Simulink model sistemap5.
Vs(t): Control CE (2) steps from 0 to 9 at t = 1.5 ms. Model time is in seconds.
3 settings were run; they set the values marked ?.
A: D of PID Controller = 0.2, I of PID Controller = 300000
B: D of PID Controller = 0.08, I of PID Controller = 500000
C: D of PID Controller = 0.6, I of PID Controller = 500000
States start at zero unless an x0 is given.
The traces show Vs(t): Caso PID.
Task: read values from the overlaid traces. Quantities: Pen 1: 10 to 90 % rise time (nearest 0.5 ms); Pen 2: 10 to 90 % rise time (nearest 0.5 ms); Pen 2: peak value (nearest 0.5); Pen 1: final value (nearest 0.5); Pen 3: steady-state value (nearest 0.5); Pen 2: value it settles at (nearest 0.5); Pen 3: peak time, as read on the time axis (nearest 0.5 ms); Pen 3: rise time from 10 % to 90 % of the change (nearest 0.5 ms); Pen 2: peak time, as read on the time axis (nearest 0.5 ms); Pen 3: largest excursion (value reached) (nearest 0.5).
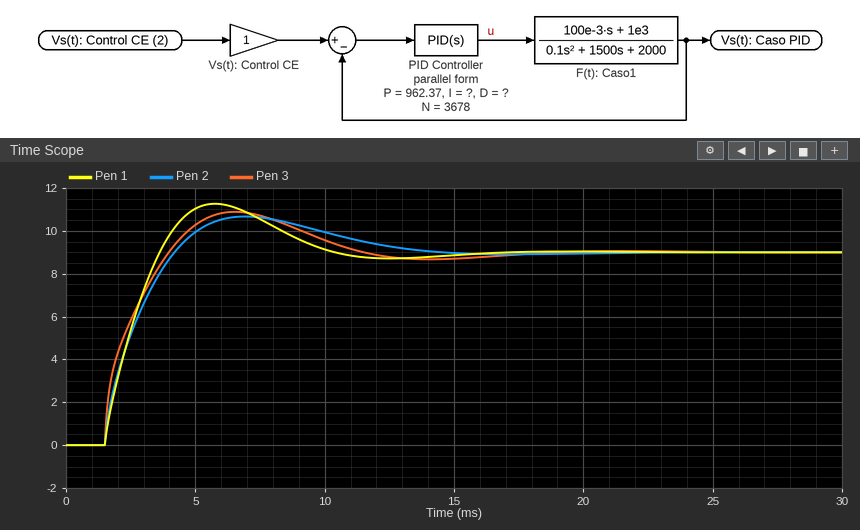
1.5 ms
2.0 ms
10.5
9.0
9.0
9.0
6.5 ms
2.0 ms
7.0 ms
11.0
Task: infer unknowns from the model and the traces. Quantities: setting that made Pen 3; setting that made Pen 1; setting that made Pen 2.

C
B
A
